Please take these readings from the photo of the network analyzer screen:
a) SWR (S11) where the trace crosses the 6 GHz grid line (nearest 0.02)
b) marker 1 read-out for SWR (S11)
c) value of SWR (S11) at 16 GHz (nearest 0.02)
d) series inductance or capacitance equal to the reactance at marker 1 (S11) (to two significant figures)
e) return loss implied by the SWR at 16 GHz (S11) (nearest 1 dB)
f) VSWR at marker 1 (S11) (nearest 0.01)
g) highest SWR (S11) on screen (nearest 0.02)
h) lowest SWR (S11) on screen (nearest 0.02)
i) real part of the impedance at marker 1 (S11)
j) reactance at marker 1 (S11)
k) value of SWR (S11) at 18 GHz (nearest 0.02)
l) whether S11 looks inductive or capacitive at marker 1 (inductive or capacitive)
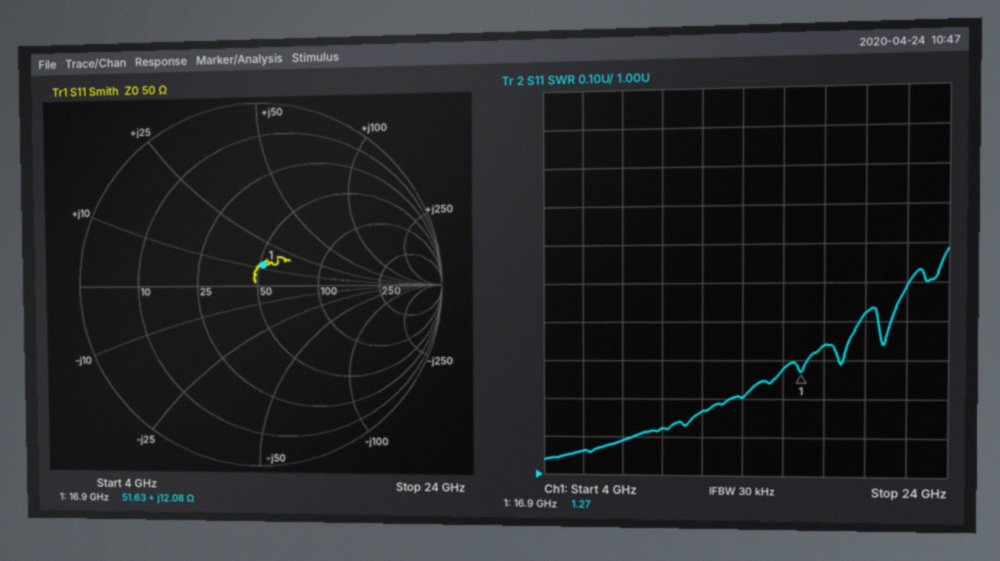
1.06
1.27
1.28
110 pH
18 dB
1.27
1.58
1.04
51.63 Ω
+12.08 Ω
1.34
inductive
